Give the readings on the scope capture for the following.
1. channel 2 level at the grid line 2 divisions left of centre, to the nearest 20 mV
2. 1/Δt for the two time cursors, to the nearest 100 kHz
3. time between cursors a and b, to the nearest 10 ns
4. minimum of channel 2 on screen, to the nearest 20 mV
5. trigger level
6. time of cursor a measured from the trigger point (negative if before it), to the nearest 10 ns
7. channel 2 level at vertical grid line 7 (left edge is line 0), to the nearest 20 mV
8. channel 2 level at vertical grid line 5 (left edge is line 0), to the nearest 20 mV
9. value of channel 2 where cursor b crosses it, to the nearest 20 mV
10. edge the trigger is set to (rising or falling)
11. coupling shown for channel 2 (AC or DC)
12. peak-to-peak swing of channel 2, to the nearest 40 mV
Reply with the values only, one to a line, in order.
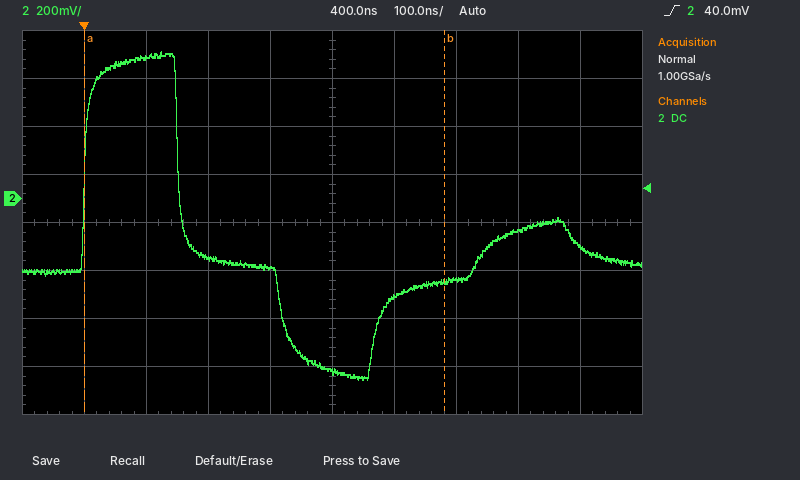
-240 mV
1.7 MHz
580 ns
-760 mV
40.0 mV
0 ns
-340 mV
-720 mV
-340 mV
rising
DC
1.36 V
